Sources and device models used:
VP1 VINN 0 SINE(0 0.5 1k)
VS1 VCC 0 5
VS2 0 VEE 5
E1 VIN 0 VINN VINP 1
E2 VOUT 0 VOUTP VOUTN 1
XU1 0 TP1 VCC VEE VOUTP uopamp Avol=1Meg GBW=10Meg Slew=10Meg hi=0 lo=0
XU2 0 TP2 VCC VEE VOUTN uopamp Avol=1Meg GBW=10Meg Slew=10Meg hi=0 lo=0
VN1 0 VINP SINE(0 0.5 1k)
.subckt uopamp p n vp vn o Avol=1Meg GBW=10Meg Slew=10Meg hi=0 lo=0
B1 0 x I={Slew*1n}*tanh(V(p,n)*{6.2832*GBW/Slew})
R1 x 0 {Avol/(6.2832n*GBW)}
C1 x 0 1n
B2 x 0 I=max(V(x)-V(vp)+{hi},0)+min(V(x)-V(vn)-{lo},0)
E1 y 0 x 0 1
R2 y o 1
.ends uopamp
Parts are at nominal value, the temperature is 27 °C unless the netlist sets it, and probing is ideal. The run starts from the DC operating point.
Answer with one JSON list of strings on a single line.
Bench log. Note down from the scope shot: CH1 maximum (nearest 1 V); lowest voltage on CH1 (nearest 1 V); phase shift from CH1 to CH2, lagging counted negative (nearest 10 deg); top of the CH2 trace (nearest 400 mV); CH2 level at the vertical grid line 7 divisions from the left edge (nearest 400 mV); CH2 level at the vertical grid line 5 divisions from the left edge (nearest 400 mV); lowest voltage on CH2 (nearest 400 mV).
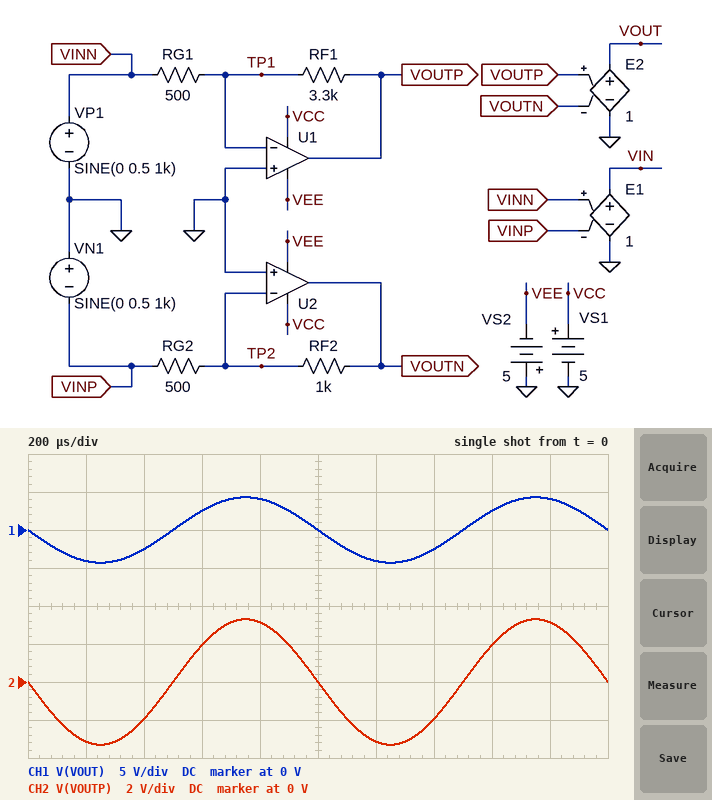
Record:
["4 V", "-4 V", "0 deg", "3.2 V", "-2.0 V", "0 V", "-3.2 V"]
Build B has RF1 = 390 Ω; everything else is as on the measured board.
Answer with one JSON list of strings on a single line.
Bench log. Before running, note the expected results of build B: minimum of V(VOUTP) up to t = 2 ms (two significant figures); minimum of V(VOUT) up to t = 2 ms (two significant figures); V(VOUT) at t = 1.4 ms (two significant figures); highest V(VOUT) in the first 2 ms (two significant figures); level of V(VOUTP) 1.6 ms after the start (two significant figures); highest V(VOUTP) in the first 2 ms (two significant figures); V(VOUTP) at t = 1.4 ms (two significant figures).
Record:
["-390 mV", "-1.4 V", "-820 mV", "1.4 V", "230 mV", "390 mV", "-230 mV"]
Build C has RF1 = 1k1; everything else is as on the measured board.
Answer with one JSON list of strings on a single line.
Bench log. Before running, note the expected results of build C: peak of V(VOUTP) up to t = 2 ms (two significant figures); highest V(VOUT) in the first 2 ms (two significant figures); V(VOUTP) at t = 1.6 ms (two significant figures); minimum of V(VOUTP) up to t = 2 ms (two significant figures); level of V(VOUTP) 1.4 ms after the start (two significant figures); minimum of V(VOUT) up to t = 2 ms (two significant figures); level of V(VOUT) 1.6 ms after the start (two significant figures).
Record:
["1.1 V", "2.1 V", "650 mV", "-1.1 V", "-650 mV", "-2.1 V", "1.2 V"]
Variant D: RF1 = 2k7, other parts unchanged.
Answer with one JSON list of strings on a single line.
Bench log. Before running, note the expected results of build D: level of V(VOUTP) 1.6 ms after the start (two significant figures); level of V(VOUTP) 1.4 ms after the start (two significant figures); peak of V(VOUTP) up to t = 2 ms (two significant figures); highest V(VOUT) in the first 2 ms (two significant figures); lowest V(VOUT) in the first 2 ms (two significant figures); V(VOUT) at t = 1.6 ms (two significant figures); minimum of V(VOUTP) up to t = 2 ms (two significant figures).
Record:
["1.6 V", "-1.6 V", "2.7 V", "3.7 V", "-3.7 V", "2.2 V", "-2.7 V"]
